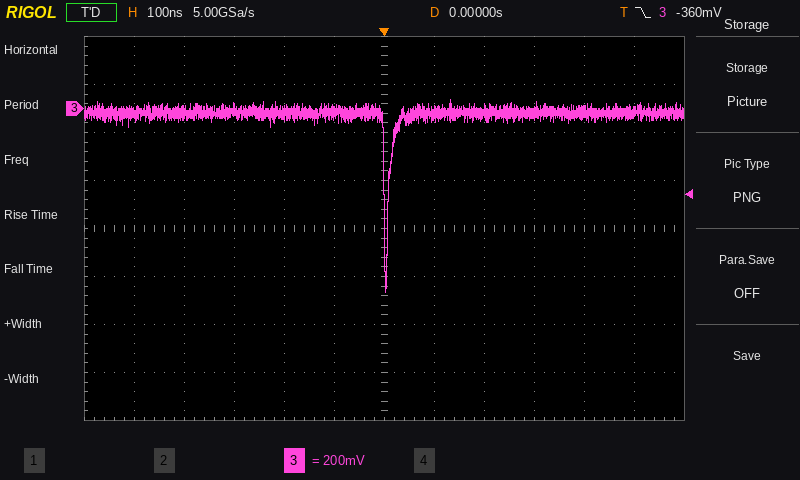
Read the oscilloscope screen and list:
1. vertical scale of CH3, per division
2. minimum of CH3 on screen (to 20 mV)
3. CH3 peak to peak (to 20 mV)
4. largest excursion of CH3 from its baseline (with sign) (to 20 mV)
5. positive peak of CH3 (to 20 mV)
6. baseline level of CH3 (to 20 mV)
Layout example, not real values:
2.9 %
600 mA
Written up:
200 mV
-760 mV
800 mV
-740 mV
40 mV
-20 mV
